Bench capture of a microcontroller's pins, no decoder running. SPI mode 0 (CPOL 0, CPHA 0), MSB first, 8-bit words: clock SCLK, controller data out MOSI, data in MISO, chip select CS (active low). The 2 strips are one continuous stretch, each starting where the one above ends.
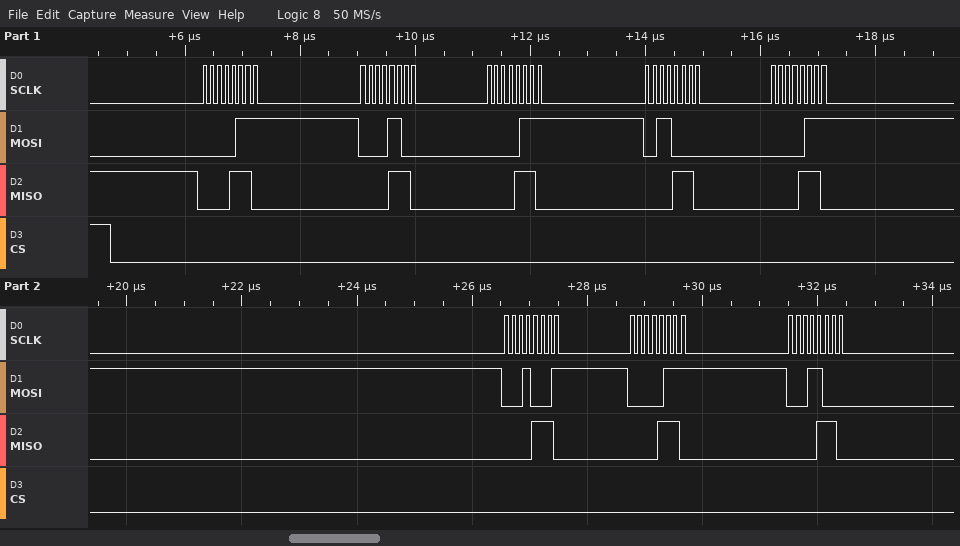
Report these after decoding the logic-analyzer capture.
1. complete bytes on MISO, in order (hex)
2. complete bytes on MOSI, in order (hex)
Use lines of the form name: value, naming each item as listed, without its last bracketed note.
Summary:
complete bytes on MISO, in order: 0E 0E 0E 0E 0E 0E 0E 0E
complete bytes on MOSI, in order: 07 0C 07 30 07 11 07 18
